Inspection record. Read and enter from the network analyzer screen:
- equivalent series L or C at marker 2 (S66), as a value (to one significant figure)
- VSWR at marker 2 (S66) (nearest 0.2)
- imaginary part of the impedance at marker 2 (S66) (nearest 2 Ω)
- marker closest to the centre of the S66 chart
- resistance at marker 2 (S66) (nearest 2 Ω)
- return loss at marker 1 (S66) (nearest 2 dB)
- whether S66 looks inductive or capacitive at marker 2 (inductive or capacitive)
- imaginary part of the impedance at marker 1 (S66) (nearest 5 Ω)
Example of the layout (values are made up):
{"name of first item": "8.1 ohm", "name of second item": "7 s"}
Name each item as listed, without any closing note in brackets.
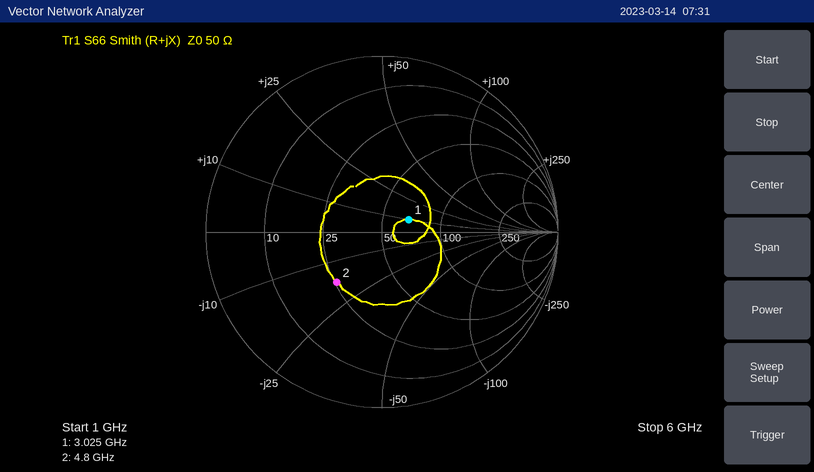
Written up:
{"equivalent series L or C at marker 2 (S66), as a value": "2 pF", "VSWR at marker 2 (S66)": "2.2", "imaginary part of the impedance at marker 2 (S66)": "-18 Ω", "marker closest to the centre of the S66 chart": "marker 1", "resistance at marker 2 (S66)": "26 Ω", "return loss at marker 1 (S66)": "16 dB", "whether S66 looks inductive or capacitive at marker 2": "capacitive", "imaginary part of the impedance at marker 1 (S66)": "+10 Ω"}
